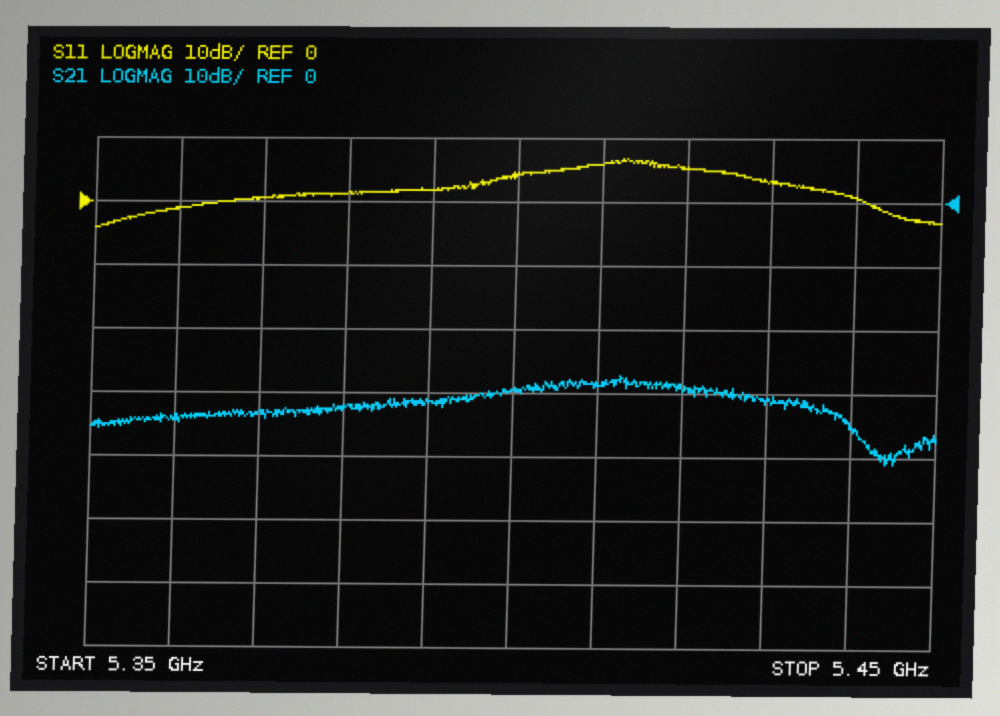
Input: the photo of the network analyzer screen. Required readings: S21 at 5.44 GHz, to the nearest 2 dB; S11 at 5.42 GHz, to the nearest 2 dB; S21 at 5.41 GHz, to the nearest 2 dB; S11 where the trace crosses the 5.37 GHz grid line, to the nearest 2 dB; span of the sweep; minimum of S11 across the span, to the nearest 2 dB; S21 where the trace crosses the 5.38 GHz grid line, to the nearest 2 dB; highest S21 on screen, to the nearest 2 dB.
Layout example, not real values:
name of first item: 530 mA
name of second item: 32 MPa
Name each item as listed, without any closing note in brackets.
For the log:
S21 at 5.44 GHz, to the nearest 2 dB: -36 dB
S11 at 5.42 GHz, to the nearest 2 dB: 6 dB
S21 at 5.41 GHz, to the nearest 2 dB: -28 dB
S11 where the trace crosses the 5.37 GHz grid line, to the nearest 2 dB: 0 dB
span of the sweep: 100 MHz
minimum of S11 across the span, to the nearest 2 dB: -4 dB
S21 where the trace crosses the 5.38 GHz grid line, to the nearest 2 dB: -32 dB
highest S21 on screen, to the nearest 2 dB: -28 dB
